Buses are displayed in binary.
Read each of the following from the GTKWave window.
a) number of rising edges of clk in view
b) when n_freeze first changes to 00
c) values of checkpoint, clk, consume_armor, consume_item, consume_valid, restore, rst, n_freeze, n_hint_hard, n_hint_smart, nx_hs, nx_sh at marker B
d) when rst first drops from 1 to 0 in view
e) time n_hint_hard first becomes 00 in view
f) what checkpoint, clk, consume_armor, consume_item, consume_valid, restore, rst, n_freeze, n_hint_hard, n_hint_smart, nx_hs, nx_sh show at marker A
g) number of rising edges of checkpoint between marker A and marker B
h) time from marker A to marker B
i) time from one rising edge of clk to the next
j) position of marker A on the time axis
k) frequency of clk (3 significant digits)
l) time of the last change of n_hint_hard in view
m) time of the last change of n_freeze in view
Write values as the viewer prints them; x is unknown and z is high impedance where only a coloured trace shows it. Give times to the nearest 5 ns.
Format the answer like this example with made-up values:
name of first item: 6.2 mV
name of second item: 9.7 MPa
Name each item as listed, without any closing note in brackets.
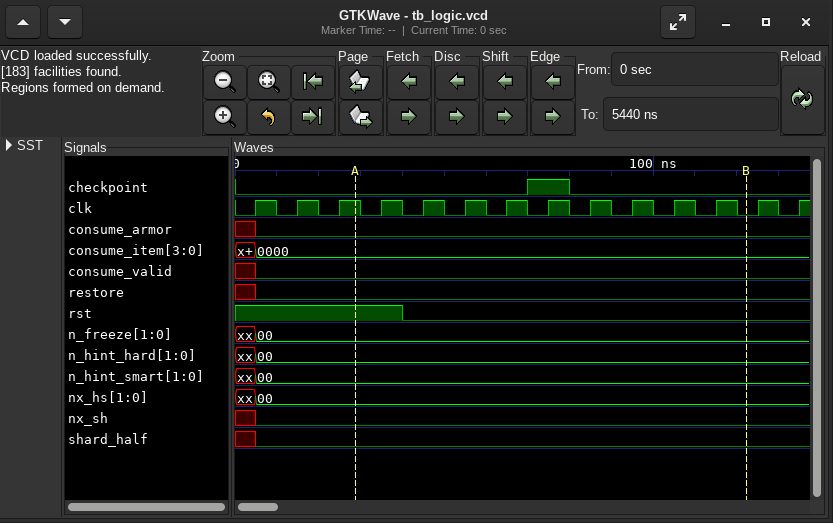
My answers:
number of rising edges of clk in view: 14
when n_freeze first changes to 00: 5 ns
values of checkpoint, clk, consume_armor, consume_item, consume_valid, restore, rst, n_freeze, n_hint_hard, n_hint_smart, nx_hs, nx_sh at marker B: checkpoint=0, clk=0, consume_armor=0, consume_item=0000, consume_valid=0, restore=0, rst=0, n_freeze=00, n_hint_hard=00, n_hint_smart=00, nx_hs=00, nx_sh=0
when rst first drops from 1 to 0 in view: 40 ns
time n_hint_hard first becomes 00 in view: 5 ns
what checkpoint, clk, consume_armor, consume_item, consume_valid, restore, rst, n_freeze, n_hint_hard, n_hint_smart, nx_hs, nx_sh show at marker A: checkpoint=0, clk=1, consume_armor=0, consume_item=0000, consume_valid=0, restore=0, rst=1, n_freeze=00, n_hint_hard=00, n_hint_smart=00, nx_hs=00, nx_sh=0
number of rising edges of checkpoint between marker A and marker B: 1
time from marker A to marker B: 95 ns
time from one rising edge of clk to the next: 10 ns
position of marker A on the time axis: 30 ns
frequency of clk: 100 MHz
time of the last change of n_hint_hard in view: 5 ns
time of the last change of n_freeze in view: 5 ns
